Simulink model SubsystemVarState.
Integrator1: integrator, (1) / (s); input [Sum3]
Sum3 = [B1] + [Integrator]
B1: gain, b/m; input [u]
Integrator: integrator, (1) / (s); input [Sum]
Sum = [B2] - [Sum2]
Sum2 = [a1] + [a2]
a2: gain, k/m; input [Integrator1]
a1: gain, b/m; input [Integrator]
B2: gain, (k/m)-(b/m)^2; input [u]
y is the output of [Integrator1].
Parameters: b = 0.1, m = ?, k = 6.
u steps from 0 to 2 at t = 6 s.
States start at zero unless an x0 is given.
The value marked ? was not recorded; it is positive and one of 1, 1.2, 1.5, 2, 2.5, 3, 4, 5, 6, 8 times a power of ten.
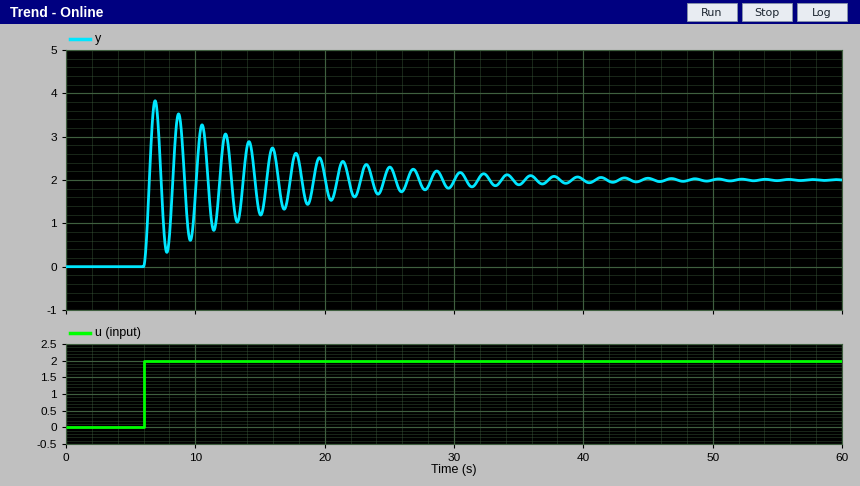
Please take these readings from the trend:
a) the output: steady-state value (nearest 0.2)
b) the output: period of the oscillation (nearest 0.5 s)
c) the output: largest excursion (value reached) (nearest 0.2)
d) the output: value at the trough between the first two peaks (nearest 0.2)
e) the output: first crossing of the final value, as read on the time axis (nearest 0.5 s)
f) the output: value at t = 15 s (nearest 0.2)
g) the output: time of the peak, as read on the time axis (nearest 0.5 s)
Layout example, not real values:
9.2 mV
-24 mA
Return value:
2.0
2.0 s
3.8
0.4
6.5 s
1.2
7.0 s
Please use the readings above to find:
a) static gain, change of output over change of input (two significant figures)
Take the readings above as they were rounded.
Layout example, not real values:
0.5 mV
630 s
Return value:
1.0
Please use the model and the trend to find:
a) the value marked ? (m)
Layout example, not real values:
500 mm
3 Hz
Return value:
0.5
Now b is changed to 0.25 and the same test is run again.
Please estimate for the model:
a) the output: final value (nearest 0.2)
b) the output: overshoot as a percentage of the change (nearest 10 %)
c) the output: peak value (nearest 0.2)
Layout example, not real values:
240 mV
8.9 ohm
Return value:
2.0
80 %
3.6
